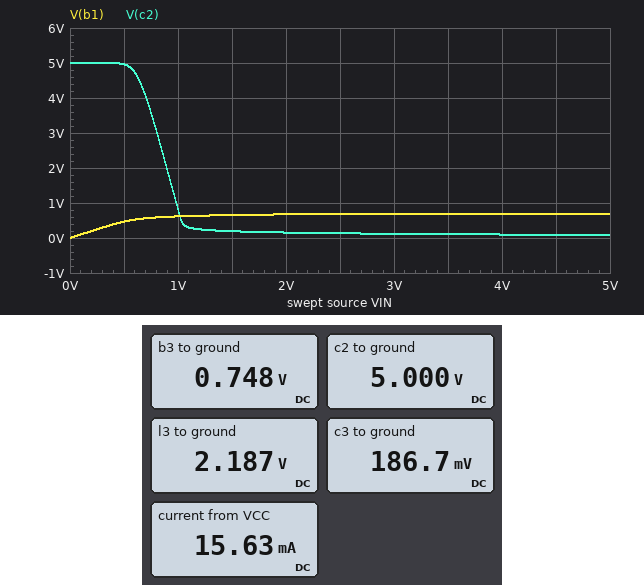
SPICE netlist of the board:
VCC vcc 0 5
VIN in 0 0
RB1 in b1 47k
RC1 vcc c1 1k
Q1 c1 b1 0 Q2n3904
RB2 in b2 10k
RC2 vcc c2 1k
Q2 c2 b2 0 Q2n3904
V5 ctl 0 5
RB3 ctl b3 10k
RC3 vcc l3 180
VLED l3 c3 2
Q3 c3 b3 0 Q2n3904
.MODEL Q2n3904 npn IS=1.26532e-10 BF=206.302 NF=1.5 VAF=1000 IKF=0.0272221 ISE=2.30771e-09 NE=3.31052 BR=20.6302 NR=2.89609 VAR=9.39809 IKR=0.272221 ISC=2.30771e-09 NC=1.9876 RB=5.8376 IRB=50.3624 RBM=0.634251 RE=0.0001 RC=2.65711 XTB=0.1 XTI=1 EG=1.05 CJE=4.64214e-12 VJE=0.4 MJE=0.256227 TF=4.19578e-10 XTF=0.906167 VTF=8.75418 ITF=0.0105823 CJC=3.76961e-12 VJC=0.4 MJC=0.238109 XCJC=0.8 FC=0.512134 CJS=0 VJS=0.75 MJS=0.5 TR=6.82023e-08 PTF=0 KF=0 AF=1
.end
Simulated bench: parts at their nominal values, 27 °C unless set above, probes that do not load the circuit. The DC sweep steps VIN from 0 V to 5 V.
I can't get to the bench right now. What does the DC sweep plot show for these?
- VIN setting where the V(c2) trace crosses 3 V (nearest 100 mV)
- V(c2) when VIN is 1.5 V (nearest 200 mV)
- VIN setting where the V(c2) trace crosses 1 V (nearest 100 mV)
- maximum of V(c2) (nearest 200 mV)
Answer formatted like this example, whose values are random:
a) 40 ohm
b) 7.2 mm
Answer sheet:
a) 800 mV
b) 200 mV
c) 1.0 V
d) 5.0 V
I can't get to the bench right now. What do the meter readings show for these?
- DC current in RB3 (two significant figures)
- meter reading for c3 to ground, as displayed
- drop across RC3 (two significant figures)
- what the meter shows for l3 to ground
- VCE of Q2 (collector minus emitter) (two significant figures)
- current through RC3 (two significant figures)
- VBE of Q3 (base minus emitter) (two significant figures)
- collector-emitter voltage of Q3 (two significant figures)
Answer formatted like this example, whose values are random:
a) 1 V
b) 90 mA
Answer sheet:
a) 430 µA
b) 186.7 mV
c) 2.8 V
d) 2.187 V
e) 5.0 V
f) 16 mA
g) 750 mV
h) 190 mV
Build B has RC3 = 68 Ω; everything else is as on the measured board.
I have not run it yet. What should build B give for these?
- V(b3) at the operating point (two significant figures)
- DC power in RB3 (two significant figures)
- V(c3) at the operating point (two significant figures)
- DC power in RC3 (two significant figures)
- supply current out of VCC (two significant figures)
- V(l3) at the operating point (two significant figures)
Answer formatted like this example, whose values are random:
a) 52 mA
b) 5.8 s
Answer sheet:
a) 790 mV
b) 1.8 mW
c) 780 mV
d) 72 mW
e) 33 mA
f) 2.8 V
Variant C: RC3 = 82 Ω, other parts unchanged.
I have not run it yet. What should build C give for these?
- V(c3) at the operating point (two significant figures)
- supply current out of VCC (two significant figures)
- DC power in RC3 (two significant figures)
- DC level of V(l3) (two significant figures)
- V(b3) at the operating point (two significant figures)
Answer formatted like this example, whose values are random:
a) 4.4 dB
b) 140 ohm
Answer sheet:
a) 410 mV
b) 32 mA
c) 82 mW
d) 2.4 V
e) 790 mV
